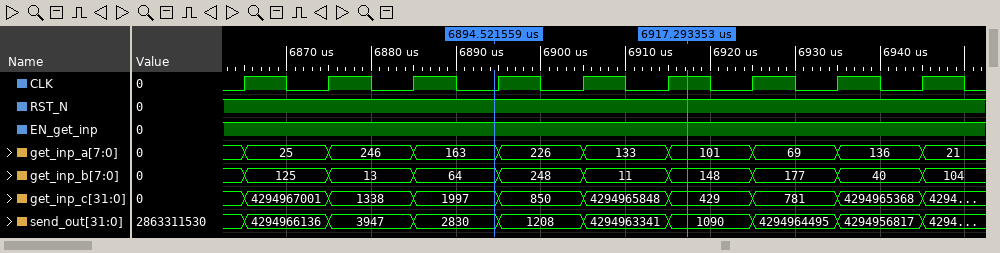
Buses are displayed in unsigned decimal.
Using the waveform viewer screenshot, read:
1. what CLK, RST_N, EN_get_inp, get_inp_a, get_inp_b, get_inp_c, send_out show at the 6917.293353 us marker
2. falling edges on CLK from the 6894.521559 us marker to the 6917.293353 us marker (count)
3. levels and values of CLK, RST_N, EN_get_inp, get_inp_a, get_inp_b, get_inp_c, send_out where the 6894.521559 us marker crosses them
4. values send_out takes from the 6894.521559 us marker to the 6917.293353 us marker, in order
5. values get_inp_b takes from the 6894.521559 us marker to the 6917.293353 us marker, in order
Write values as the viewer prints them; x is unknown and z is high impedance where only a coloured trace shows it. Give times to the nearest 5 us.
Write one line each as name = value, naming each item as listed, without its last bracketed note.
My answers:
what CLK, RST_N, EN_get_inp, get_inp_a, get_inp_b, get_inp_c, send_out show at the 6917.293353 us marker = CLK=1, RST_N=1, EN_get_inp=1, get_inp_a=101, get_inp_b=148, get_inp_c=429, send_out=1090
falling edges on CLK from the 6894.521559 us marker to the 6917.293353 us marker = 2
levels and values of CLK, RST_N, EN_get_inp, get_inp_a, get_inp_b, get_inp_c, send_out where the 6894.521559 us marker crosses them = CLK=0, RST_N=1, EN_get_inp=1, get_inp_a=163, get_inp_b=64, get_inp_c=1997, send_out=2830
values send_out takes from the 6894.521559 us marker to the 6917.293353 us marker, in order = 2830, 1208, 4294963341, 1090
values get_inp_b takes from the 6894.521559 us marker to the 6917.293353 us marker, in order = 64, 248, 11, 148
